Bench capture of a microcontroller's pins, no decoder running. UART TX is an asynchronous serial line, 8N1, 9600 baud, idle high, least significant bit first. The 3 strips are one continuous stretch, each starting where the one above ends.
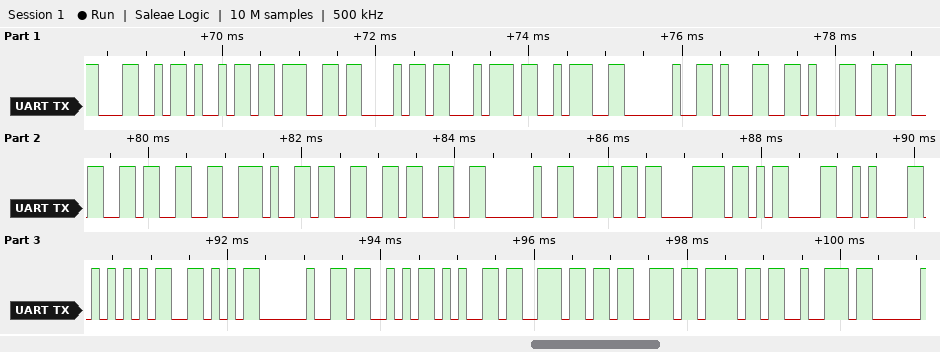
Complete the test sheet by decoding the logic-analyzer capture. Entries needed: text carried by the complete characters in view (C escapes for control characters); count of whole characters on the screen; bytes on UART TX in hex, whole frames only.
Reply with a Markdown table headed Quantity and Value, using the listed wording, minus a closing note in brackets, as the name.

| Quantity | Value |
|---|---|
| text carried by the complete characters in view | "Light: 1133.33 lx\r\nUV Sensor" |
| count of whole characters on the screen | 28 |
| bytes on UART TX in hex, whole frames only | 0x4C 0x69 0x67 0x68 0x74 0x3A 0x20 0x31 0x31 0x33 0x33 0x2E 0x33 0x33 0x20 0x6C 0x78 0x0D 0x0A 0x55 0x56 0x20 0x53 0x65 0x6E 0x73 0x6F 0x72 |
